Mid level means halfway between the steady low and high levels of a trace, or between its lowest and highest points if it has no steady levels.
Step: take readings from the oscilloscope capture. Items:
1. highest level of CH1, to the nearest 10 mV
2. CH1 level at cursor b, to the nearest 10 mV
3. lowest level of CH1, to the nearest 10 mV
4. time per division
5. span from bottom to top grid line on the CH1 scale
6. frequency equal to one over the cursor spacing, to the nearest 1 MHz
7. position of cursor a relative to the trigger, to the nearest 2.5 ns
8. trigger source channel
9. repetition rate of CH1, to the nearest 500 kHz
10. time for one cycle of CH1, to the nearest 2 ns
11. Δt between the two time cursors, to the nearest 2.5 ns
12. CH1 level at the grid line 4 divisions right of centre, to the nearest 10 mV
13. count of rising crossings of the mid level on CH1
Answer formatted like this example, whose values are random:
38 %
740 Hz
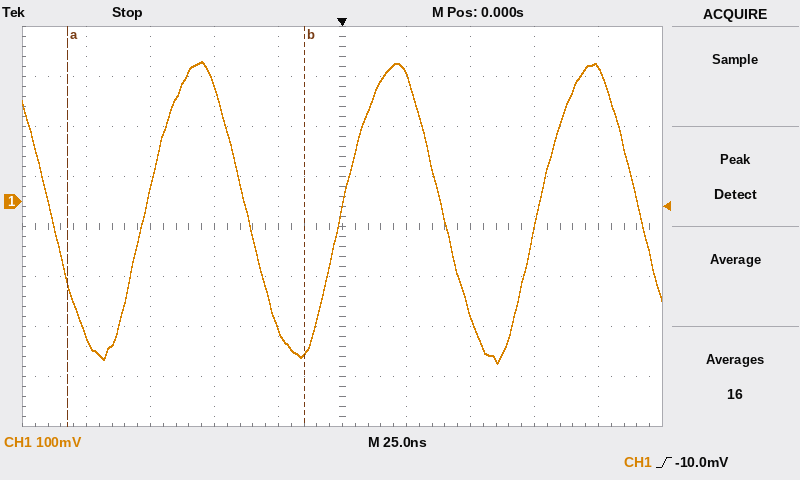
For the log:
280 mV
-300 mV
-320 mV
25 ns
800 mV
11 MHz
-107.5 ns
CH1
13.0 MHz
76 ns
92.5 ns
270 mV
3
